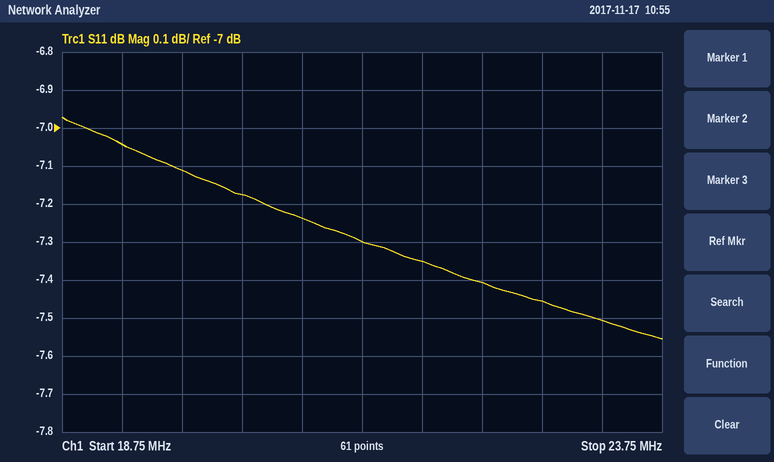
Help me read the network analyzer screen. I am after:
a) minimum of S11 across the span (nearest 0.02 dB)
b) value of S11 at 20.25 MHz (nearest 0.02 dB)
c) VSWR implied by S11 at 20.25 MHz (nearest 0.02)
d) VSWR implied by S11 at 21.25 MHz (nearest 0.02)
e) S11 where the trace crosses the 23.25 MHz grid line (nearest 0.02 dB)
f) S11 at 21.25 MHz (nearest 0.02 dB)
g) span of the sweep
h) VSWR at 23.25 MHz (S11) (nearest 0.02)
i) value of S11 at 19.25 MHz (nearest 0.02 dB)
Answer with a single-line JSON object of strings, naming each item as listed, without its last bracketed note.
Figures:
{"minimum of S11 across the span": "-7.56 dB", "value of S11 at 20.25 MHz": "-7.18 dB", "VSWR implied by S11 at 20.25 MHz": "2.56", "VSWR implied by S11 at 21.25 MHz": "2.52", "S11 where the trace crosses the 23.25 MHz grid line": "-7.50 dB", "S11 at 21.25 MHz": "-7.30 dB", "span of the sweep": "5 MHz", "VSWR at 23.25 MHz (S11)": "2.46", "value of S11 at 19.25 MHz": "-7.04 dB"}
